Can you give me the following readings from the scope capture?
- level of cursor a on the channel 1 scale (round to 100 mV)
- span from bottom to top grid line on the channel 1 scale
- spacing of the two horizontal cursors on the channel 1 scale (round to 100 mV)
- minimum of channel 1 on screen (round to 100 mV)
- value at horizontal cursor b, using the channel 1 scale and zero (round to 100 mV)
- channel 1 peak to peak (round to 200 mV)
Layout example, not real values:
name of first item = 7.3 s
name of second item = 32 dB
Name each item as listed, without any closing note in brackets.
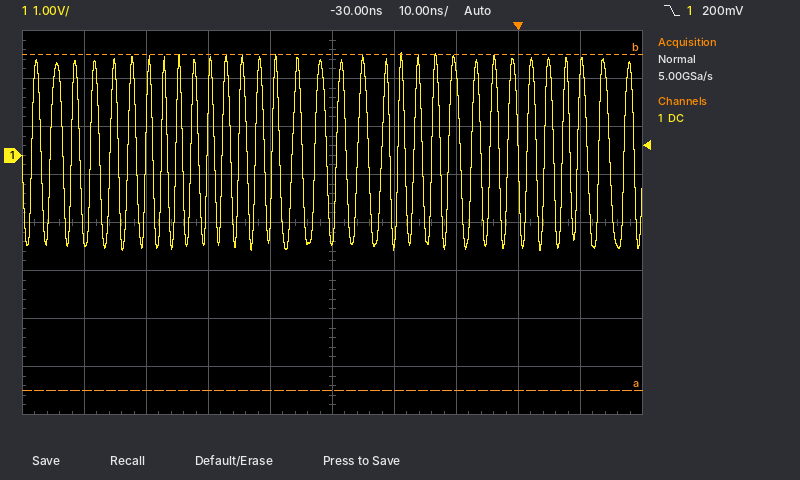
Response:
level of cursor a on the channel 1 scale = -4.9 V
span from bottom to top grid line on the channel 1 scale = 8 V
spacing of the two horizontal cursors on the channel 1 scale = 7.0 V
minimum of channel 1 on screen = -2.0 V
value at horizontal cursor b, using the channel 1 scale and zero = 2.1 V
channel 1 peak to peak = 4.2 V
